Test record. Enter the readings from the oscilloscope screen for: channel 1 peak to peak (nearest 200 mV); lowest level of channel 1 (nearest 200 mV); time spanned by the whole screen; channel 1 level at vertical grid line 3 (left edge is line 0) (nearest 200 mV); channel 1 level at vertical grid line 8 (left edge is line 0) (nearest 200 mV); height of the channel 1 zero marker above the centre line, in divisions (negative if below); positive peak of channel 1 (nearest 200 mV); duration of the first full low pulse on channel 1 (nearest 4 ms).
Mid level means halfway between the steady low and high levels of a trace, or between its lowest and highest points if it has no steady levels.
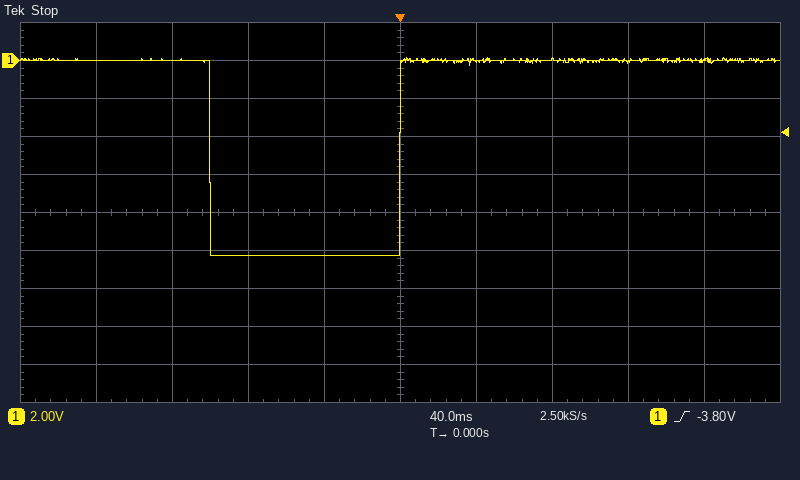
10.4 V
-10.2 V
400 ms
-10.2 V
0.0 V
+4.0 div
200 mV
100 ms
